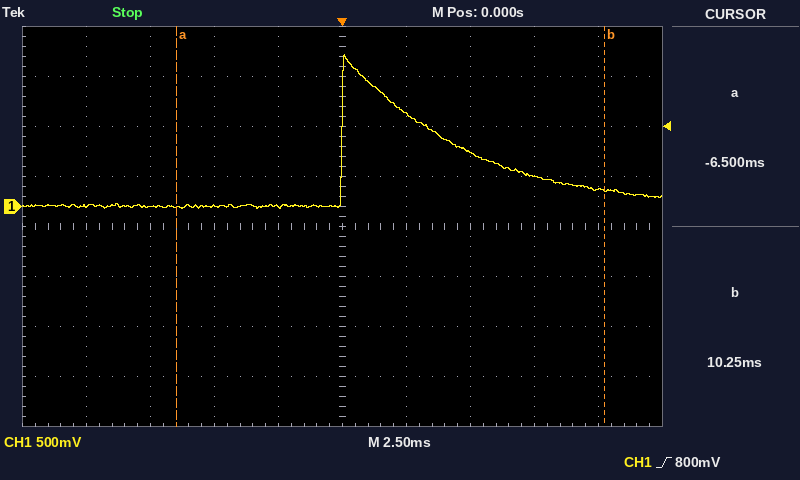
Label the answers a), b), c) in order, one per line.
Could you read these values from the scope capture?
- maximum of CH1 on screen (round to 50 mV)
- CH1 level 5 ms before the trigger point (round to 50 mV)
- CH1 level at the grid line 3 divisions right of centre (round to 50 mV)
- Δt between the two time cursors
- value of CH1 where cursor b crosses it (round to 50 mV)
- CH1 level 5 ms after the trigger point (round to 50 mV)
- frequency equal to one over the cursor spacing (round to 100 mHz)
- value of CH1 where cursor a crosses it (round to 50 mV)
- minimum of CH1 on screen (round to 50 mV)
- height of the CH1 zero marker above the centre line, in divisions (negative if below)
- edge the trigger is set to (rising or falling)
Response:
a) 1.50 V
b) 0 mV
c) 300 mV
d) 16.75 ms
e) 150 mV
f) 550 mV
g) 59.7 Hz
h) 0 mV
i) 0 mV
j) +0.4 div
k) rising
